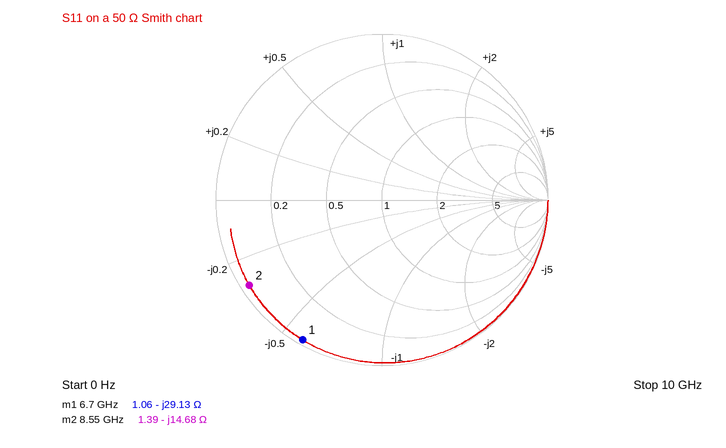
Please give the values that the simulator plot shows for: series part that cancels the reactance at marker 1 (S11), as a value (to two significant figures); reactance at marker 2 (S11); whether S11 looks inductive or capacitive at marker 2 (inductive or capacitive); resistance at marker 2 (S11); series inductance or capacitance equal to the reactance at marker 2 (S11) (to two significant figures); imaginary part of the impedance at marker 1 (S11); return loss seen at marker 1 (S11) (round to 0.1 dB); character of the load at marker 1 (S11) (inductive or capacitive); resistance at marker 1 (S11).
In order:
690 pH
-14.68 Ω
capacitive
1.39 Ω
1.3 pF
-29.13 Ω
0.3 dB
capacitive
1.06 Ω
